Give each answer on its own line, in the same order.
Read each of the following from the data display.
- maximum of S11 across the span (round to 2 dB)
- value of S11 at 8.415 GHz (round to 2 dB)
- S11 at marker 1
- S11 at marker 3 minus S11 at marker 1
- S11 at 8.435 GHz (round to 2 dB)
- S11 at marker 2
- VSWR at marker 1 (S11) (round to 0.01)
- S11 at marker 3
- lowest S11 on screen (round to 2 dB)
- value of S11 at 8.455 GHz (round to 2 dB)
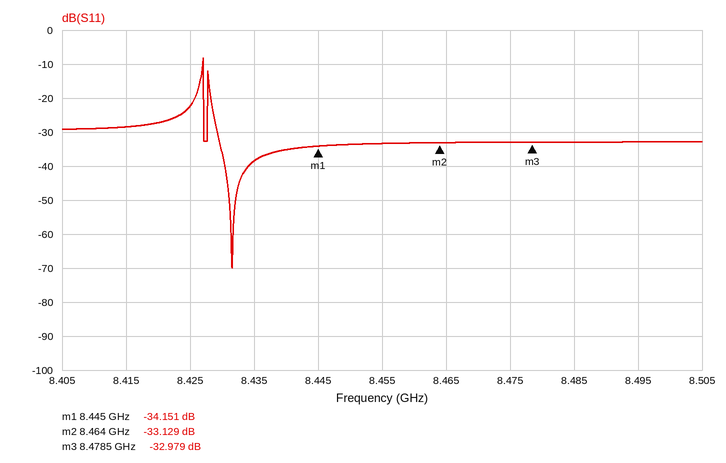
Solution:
-8 dB
-28 dB
-34.151 dB
1.172 dB
-38 dB
-33.129 dB
1.04
-32.979 dB
-70 dB
-34 dB
